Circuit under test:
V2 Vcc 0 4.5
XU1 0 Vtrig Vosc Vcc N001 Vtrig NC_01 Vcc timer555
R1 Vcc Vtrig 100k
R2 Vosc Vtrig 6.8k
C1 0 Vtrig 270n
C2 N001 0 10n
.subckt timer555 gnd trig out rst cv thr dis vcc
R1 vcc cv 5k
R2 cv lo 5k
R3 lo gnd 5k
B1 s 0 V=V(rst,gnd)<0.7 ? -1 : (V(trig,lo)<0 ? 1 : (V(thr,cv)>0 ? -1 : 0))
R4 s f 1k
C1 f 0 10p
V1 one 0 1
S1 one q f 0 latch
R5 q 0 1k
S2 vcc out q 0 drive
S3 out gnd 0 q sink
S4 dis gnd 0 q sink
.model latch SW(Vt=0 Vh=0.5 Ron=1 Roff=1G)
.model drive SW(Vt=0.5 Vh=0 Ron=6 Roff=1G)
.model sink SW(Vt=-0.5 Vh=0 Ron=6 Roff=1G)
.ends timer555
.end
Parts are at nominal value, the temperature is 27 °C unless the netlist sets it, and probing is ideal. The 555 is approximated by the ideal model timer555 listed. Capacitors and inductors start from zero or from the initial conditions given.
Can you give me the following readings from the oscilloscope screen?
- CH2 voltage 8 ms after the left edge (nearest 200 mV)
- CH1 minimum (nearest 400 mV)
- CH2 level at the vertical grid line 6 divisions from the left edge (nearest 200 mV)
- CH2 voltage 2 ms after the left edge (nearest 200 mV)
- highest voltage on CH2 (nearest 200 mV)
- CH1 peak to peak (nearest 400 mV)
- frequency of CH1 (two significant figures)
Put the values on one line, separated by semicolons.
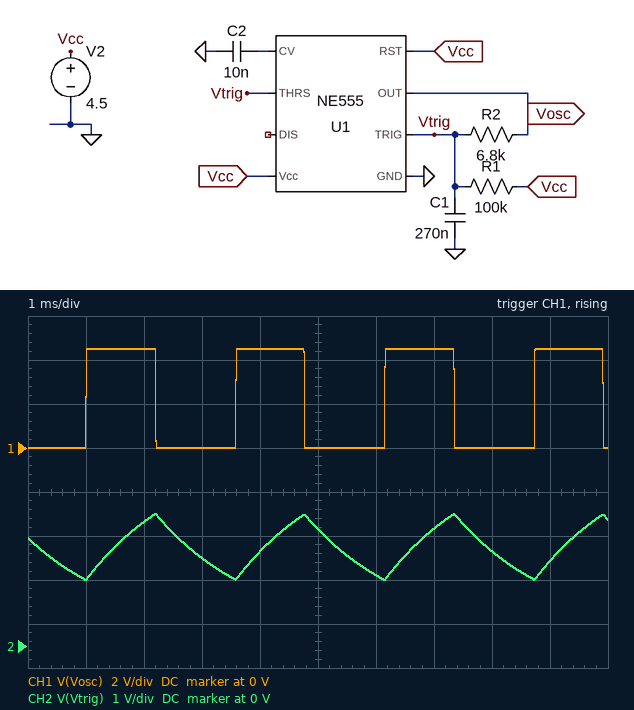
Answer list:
2.2 V; 0 V; 1.6 V; 2.8 V; 3.0 V; 4.4 V; 390 Hz
